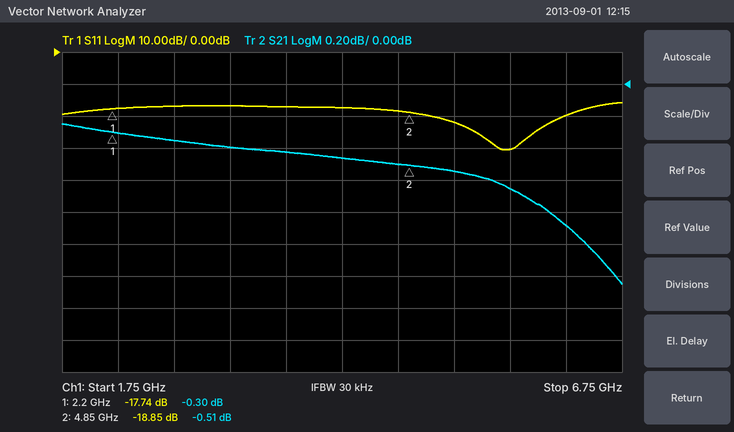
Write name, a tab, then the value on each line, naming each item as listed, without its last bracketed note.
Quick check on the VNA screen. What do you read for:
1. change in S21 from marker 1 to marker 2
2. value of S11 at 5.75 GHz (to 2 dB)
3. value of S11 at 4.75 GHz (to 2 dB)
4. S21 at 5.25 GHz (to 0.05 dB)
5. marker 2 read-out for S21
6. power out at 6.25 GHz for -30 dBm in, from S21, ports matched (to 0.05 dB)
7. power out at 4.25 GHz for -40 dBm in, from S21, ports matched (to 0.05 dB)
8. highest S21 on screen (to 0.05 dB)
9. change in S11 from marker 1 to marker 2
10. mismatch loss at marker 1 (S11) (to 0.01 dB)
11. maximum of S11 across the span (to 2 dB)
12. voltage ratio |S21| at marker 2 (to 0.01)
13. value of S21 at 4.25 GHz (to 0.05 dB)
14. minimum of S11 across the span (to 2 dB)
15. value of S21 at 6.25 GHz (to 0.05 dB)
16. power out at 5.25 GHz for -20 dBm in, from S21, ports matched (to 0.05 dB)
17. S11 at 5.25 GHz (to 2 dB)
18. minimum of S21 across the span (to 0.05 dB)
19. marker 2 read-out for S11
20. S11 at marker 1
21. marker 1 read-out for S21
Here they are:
change in S21 from marker 1 to marker 2	-0.21 dB
value of S11 at 5.75 GHz	-30 dB
value of S11 at 4.75 GHz	-18 dB
S21 at 5.25 GHz	-0.55 dB
marker 2 read-out for S21	-0.51 dB
power out at 6.25 GHz for -30 dBm in, from S21, ports matched	-30.90 dBm
power out at 4.25 GHz for -40 dBm in, from S21, ports matched	-40.45 dBm
highest S21 on screen	-0.25 dB
change in S11 from marker 1 to marker 2	-1.11 dB
mismatch loss at marker 1 (S11)	0.07 dB
maximum of S11 across the span	-16 dB
voltage ratio |S21| at marker 2	0.94
value of S21 at 4.25 GHz	-0.45 dB
minimum of S11 across the span	-30 dB
value of S21 at 6.25 GHz	-0.90 dB
power out at 5.25 GHz for -20 dBm in, from S21, ports matched	-20.55 dBm
S11 at 5.25 GHz	-22 dB
minimum of S21 across the span	-1.25 dB
marker 2 read-out for S11	-18.85 dB
S11 at marker 1	-17.74 dB
marker 1 read-out for S21	-0.30 dB
